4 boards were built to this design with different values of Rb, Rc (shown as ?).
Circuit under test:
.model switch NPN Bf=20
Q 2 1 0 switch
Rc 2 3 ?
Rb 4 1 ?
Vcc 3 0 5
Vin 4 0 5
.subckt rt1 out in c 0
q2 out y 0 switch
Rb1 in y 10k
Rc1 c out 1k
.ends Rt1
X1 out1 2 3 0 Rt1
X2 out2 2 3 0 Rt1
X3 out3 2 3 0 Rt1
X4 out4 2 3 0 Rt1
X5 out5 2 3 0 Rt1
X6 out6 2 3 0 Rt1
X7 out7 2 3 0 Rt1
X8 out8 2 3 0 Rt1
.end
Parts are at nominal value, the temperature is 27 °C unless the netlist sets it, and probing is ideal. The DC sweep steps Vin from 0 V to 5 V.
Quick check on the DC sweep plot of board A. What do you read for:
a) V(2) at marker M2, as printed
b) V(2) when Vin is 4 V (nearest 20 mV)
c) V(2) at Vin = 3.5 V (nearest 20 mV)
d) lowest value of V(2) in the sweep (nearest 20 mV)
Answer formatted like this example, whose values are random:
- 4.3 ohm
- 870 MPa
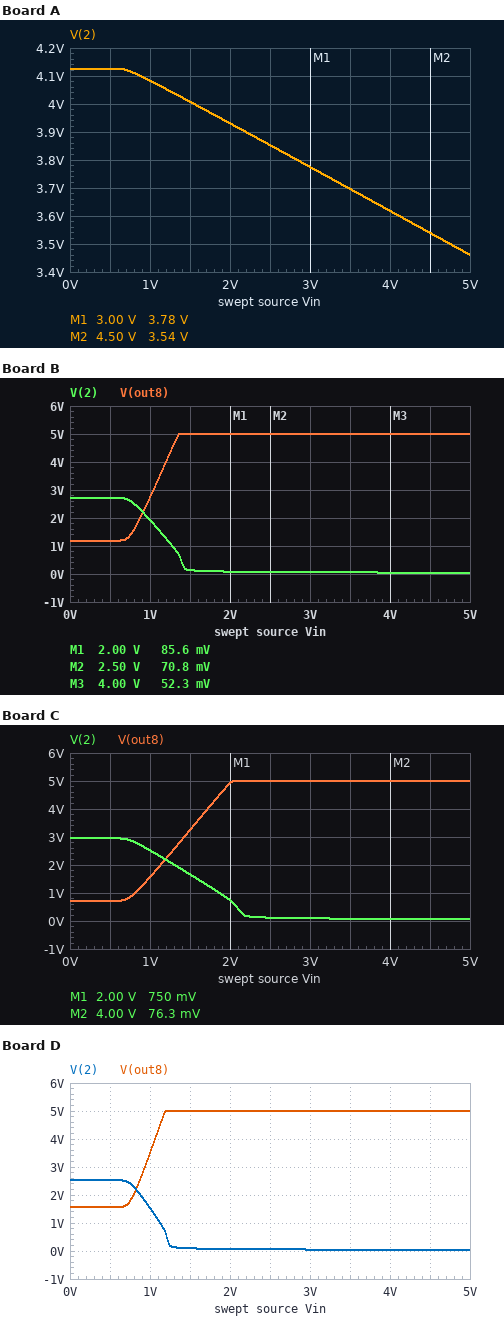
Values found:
- 3.54 V
- 3.62 V
- 3.70 V
- 3.46 V
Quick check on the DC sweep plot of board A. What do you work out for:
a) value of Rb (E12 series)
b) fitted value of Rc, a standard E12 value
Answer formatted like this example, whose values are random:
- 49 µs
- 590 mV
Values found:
- 33 kΩ
- 330 Ω
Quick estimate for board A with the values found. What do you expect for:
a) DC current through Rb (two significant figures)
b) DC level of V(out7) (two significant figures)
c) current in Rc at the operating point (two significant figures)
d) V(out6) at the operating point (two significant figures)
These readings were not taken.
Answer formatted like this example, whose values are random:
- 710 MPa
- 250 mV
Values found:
- 130 µA
- 140 mV
- 4.7 mA
- 140 mV
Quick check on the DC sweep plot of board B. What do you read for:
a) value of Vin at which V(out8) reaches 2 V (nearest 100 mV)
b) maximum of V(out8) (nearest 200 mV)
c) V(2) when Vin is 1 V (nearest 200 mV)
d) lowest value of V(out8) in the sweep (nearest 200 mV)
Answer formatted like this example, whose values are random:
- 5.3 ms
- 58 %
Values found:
- 900 mV
- 5.0 V
- 2.0 V
- 1.2 V
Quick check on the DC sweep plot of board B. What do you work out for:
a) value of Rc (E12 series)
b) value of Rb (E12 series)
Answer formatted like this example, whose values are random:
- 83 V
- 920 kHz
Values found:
- 1.5 kΩ
- 3.9 kΩ
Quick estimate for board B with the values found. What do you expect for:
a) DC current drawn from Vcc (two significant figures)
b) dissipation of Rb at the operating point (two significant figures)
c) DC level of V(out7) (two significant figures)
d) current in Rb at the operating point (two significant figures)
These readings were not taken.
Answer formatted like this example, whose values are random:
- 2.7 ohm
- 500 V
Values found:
- 3.3 mA
- 4.5 mW
- 5.0 V
- 1.1 mA
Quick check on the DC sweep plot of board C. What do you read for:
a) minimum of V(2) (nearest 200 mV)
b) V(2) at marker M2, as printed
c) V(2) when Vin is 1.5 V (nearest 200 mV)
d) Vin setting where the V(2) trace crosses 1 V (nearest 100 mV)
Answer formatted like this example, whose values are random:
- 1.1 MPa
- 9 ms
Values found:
- 0 V
- 76.3 mV
- 1.6 V
- 1.9 V
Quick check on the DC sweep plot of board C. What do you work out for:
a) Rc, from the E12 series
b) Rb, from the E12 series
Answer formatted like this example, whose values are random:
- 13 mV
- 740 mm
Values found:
- 1.2 kΩ
- 6.8 kΩ
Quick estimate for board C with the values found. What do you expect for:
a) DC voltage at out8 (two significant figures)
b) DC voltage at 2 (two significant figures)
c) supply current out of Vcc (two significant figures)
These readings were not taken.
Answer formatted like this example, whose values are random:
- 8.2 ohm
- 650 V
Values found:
- 5.0 V
- 66 mV
- 4.1 mA
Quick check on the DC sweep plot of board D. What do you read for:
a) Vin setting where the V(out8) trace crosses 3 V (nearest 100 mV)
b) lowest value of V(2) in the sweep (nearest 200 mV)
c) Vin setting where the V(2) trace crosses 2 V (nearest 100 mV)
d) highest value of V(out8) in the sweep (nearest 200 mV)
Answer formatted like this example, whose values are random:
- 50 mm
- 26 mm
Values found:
- 900 mV
- 0 V
- 900 mV
- 5.0 V
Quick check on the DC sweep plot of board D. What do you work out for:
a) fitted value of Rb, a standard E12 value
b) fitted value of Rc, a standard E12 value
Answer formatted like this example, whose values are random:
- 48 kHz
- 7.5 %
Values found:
- 3.3 kΩ
- 1.8 kΩ
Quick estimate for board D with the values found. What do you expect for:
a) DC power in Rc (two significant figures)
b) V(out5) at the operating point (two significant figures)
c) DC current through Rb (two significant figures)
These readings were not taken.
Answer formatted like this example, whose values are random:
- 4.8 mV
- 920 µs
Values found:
- 14 mW
- 5.0 V
- 1.3 mA
